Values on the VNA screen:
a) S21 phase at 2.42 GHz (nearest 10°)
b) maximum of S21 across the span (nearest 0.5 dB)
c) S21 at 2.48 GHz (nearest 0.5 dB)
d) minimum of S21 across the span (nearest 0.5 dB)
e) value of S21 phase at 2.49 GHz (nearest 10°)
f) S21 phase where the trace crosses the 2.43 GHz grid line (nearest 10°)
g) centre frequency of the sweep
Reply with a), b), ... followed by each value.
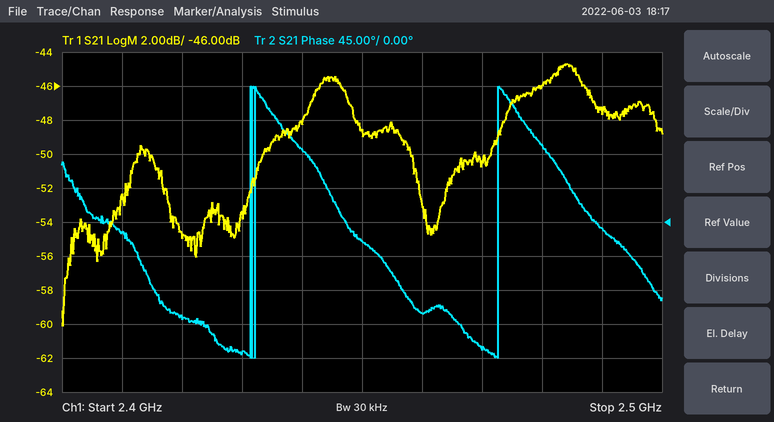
a) -130°
b) -44.5 dB
c) -46.0 dB
d) -60.0 dB
e) -10°
f) -170°
g) 2.45 GHz
